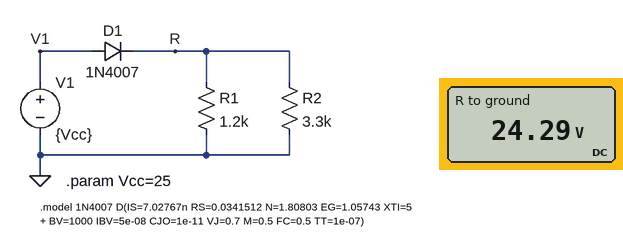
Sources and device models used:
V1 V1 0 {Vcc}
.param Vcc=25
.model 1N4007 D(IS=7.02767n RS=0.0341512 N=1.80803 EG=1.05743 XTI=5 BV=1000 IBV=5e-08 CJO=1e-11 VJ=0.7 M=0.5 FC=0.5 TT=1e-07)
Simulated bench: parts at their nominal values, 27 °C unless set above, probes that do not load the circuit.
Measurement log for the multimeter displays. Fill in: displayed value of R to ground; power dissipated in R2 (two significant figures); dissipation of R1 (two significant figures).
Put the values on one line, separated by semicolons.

24.29 V; 180 mW; 490 mW
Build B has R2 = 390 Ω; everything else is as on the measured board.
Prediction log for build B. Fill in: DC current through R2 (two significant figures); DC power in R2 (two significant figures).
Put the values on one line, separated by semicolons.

62 mA; 1.5 W
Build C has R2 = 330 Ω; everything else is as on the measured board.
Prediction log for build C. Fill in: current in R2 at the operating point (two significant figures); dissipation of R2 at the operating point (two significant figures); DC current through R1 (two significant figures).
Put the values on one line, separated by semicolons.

73 mA; 1.8 W; 20 mA
